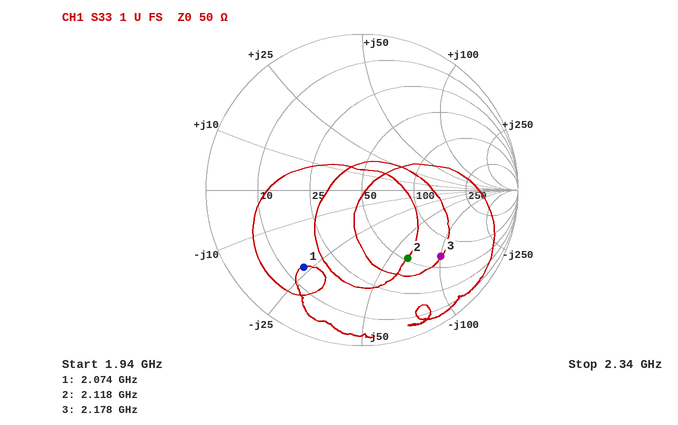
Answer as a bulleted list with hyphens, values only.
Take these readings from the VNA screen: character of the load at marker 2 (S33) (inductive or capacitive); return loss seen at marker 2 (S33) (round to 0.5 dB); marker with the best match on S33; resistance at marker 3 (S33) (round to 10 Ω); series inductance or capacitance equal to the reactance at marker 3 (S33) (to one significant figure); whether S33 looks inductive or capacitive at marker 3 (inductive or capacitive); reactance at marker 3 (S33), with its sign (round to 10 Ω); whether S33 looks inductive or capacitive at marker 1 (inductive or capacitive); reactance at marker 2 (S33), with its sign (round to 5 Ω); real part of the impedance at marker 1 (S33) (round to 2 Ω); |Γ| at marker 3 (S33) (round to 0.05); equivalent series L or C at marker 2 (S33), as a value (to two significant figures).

- capacitive
- 5.5 dB
- marker 2
- 70 Ω
- 700 fF
- capacitive
- -100 Ω
- capacitive
- -65 Ω
- 14 Ω
- 0.65
- 1.2 pF
